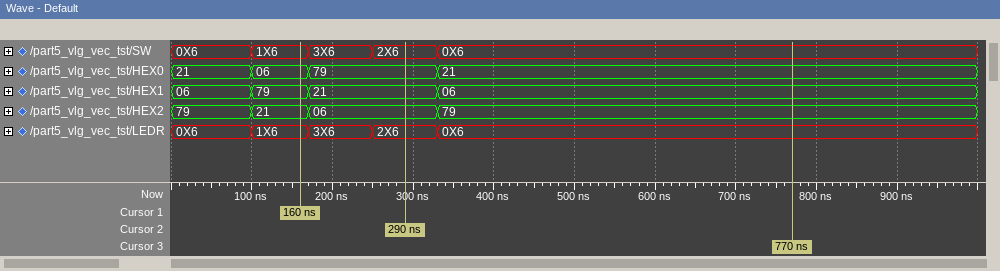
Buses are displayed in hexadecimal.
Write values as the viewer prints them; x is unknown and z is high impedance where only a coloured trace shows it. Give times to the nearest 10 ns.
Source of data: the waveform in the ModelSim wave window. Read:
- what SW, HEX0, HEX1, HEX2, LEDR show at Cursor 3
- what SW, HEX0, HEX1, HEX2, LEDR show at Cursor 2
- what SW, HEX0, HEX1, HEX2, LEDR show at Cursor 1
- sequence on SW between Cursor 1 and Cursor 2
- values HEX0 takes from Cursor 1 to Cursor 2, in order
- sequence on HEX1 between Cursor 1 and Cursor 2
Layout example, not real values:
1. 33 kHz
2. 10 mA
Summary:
1. SW=0X6, HEX0=21, HEX1=06, HEX2=79, LEDR=0X6
2. SW=2X6, HEX0=79, HEX1=21, HEX2=06, LEDR=2X6
3. SW=1X6, HEX0=06, HEX1=79, HEX2=21, LEDR=1X6
4. 1X6, 3X6, 2X6
5. 06, 79
6. 79, 21
